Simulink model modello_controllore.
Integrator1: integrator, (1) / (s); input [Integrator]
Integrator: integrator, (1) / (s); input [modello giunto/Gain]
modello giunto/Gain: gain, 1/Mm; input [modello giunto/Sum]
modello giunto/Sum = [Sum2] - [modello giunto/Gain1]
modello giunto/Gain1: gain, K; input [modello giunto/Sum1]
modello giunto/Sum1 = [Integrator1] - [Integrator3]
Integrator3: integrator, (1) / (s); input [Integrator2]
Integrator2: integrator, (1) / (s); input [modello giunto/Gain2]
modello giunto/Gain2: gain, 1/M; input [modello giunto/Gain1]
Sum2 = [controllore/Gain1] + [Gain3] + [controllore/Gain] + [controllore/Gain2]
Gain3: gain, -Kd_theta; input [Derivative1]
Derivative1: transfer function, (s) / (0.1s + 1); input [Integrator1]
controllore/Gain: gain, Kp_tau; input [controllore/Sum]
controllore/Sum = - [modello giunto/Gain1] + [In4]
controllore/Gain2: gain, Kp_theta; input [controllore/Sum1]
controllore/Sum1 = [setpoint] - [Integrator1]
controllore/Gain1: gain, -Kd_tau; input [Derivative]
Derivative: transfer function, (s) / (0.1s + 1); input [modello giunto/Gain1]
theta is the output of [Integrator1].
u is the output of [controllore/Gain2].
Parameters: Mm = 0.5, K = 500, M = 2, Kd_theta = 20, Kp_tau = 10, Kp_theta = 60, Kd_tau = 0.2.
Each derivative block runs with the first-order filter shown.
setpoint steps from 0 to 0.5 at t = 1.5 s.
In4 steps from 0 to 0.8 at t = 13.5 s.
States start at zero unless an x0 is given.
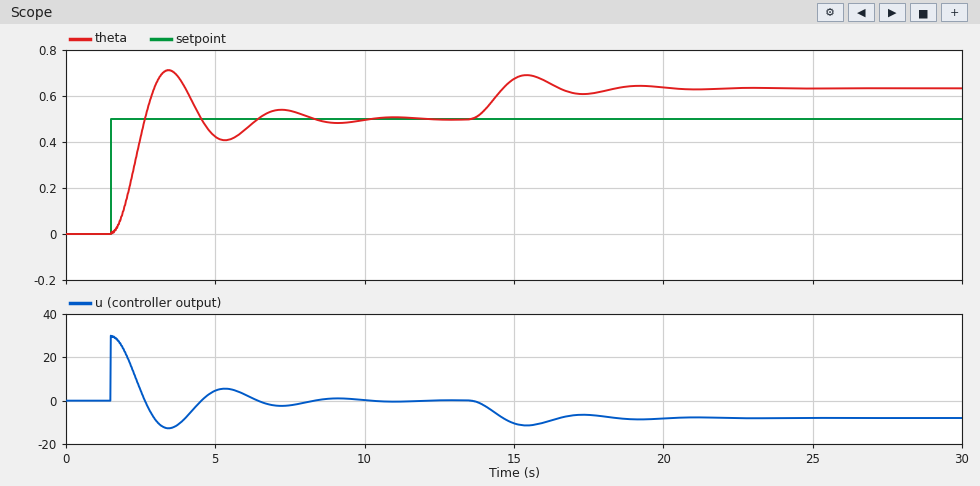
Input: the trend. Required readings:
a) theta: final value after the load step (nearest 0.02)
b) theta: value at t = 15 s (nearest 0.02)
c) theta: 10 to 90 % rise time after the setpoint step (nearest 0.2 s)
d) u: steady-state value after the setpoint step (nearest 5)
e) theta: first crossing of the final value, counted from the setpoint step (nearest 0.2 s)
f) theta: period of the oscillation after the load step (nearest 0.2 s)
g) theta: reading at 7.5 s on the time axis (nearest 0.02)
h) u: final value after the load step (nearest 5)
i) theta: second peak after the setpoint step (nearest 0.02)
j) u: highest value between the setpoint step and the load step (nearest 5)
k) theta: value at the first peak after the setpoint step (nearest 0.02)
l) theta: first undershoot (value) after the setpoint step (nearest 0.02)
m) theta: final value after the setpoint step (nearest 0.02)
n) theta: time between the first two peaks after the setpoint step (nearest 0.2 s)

0.64
0.68
0.8 s
0
1.2 s
3.8 s
0.54
-10
0.54
30
0.72
0.40
0.50
3.8 s
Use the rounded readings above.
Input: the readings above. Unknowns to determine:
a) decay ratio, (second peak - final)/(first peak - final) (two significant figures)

0.18
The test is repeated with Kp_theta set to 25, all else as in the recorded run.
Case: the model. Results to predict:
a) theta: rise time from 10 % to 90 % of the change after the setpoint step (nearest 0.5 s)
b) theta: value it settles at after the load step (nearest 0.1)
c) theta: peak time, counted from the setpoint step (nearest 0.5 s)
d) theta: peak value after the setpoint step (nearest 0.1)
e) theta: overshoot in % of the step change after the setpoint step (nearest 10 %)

1.5 s
0.8
3.0 s
0.6
20 %
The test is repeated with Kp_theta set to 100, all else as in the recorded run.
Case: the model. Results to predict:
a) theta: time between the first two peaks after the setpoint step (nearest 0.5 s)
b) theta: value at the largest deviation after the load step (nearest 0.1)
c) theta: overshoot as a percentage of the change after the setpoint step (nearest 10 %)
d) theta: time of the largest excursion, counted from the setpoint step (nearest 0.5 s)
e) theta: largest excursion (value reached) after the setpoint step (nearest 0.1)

3.0 s
0.6
50 %
1.5 s
0.8
